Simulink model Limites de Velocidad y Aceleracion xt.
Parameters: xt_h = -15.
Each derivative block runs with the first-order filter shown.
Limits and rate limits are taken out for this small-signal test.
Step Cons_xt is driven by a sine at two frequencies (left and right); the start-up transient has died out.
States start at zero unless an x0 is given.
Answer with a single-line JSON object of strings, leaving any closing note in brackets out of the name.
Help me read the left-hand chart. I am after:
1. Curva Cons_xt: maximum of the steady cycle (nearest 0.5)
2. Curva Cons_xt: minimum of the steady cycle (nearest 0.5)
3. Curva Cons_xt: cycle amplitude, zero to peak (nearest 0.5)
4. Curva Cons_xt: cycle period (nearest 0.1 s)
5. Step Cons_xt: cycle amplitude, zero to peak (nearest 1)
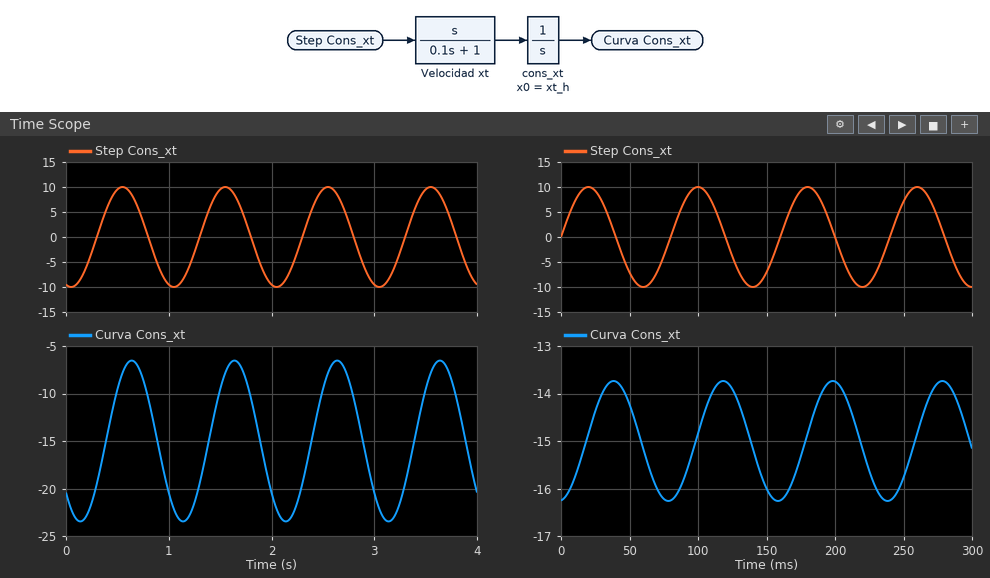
{"Curva Cons_xt: maximum of the steady cycle": "-6.5", "Curva Cons_xt: minimum of the steady cycle": "-23.5", "Curva Cons_xt: cycle amplitude, zero to peak": "8.5", "Curva Cons_xt: cycle period": "1.0 s", "Step Cons_xt: cycle amplitude, zero to peak": "10"}
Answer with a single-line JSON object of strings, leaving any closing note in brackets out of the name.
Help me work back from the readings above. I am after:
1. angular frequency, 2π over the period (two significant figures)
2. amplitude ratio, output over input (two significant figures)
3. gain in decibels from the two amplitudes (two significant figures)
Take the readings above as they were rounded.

{"angular frequency, 2π over the period": "6.3 rad/s", "amplitude ratio, output over input": "0.85", "gain in decibels from the two amplitudes": "-1.4 dB"}
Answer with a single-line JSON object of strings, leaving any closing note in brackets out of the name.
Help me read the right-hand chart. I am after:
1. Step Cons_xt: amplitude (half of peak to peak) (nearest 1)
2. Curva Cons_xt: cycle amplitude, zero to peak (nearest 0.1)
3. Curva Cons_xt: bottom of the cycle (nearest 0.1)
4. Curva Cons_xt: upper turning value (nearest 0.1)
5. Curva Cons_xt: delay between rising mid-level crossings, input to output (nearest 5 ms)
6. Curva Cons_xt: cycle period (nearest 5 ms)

{"Step Cons_xt: amplitude (half of peak to peak)": "10", "Curva Cons_xt: cycle amplitude, zero to peak": "1.3", "Curva Cons_xt: bottom of the cycle": "-16.3", "Curva Cons_xt: upper turning value": "-13.7", "Curva Cons_xt: delay between rising mid-level crossings, input to output": "20 ms", "Curva Cons_xt: cycle period": "80 ms"}
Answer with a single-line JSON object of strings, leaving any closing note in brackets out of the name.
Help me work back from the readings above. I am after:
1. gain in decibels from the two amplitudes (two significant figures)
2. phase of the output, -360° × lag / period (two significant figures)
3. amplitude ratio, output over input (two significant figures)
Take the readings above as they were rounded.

{"gain in decibels from the two amplitudes": "-18 dB", "phase of the output, -360° × lag / period": "-90°", "amplitude ratio, output over input": "0.13"}
